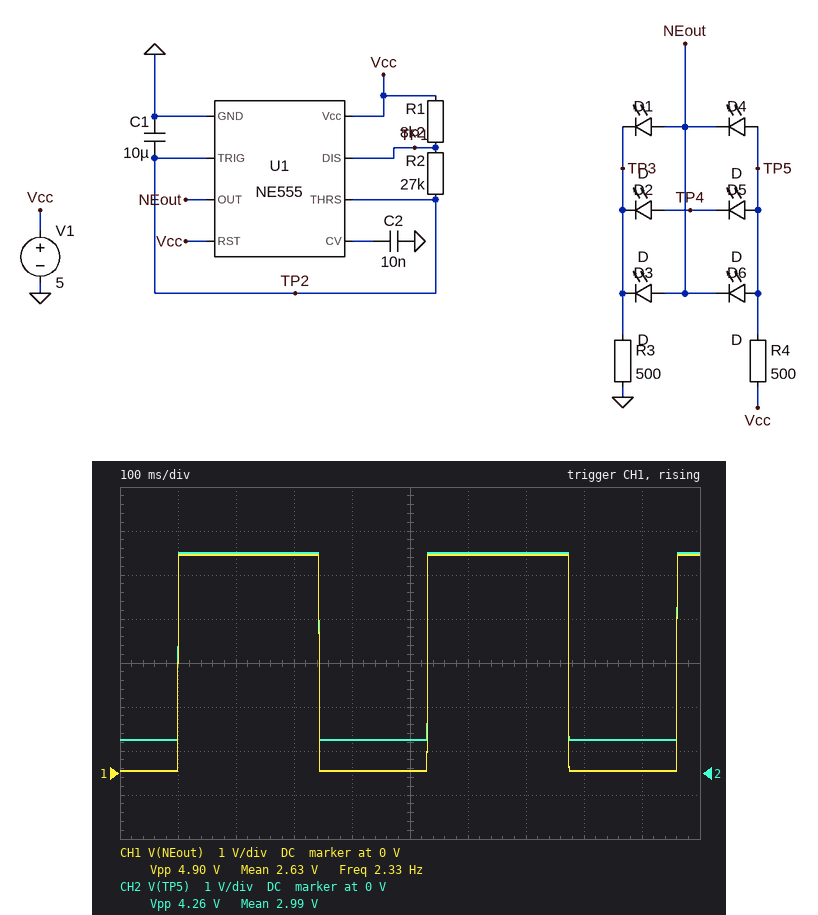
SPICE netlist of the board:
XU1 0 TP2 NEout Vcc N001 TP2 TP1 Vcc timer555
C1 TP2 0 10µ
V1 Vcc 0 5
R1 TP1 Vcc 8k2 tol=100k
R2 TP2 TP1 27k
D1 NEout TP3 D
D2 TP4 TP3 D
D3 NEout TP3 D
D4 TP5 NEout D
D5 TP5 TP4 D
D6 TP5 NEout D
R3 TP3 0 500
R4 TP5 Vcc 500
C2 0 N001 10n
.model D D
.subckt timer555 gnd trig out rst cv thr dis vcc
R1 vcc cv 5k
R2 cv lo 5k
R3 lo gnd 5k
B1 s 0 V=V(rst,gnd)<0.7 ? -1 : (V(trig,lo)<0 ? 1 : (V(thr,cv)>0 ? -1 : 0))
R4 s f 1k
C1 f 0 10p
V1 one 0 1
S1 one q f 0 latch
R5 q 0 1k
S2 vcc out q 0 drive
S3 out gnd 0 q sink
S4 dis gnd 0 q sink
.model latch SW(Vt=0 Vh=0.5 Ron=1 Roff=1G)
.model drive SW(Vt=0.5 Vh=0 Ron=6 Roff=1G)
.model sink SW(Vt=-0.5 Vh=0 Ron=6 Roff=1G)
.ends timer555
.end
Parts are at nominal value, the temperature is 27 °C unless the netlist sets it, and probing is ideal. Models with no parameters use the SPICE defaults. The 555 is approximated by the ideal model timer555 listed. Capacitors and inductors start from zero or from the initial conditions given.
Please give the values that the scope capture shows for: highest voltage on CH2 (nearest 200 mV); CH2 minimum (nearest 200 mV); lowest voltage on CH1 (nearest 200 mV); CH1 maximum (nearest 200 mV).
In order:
5.0 V
800 mV
0 V
5.0 V
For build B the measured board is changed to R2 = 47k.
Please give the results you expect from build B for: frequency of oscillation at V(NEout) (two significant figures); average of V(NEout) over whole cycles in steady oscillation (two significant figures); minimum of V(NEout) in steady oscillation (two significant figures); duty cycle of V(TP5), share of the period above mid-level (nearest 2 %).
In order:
1.4 Hz
2.7 V
51 mV
54 %
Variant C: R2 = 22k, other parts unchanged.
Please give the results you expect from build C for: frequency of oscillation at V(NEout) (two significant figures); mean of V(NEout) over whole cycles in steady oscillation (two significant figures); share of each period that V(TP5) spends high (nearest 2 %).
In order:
2.8 Hz
2.9 V
58 %
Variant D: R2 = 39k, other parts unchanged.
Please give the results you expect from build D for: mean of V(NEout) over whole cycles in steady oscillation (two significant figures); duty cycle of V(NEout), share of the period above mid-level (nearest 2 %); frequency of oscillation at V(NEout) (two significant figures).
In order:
2.7 V
54 %
1.7 Hz
